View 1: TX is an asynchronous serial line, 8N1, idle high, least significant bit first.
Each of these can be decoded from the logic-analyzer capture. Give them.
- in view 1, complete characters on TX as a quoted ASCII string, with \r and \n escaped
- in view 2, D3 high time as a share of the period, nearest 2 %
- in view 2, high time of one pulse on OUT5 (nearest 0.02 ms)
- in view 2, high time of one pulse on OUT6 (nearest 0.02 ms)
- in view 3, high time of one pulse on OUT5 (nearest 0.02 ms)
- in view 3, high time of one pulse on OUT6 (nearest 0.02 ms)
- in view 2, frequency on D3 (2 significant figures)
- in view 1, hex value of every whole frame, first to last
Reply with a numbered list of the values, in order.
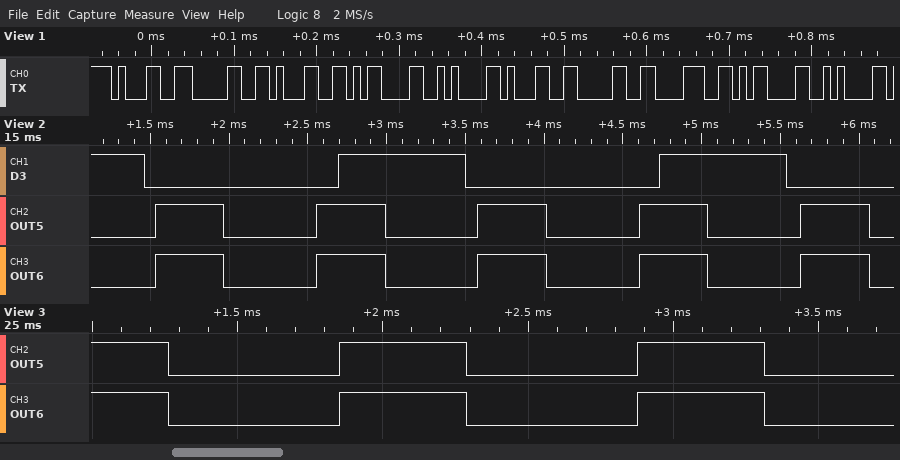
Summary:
1. "101\r\n108\r\n"
2. 40 %
3. 0.44 ms
4. 0.44 ms
5. 0.44 ms
6. 0.44 ms
7. 490 Hz
8. 31 30 31 0D 0A 31 30 38 0D 0A
